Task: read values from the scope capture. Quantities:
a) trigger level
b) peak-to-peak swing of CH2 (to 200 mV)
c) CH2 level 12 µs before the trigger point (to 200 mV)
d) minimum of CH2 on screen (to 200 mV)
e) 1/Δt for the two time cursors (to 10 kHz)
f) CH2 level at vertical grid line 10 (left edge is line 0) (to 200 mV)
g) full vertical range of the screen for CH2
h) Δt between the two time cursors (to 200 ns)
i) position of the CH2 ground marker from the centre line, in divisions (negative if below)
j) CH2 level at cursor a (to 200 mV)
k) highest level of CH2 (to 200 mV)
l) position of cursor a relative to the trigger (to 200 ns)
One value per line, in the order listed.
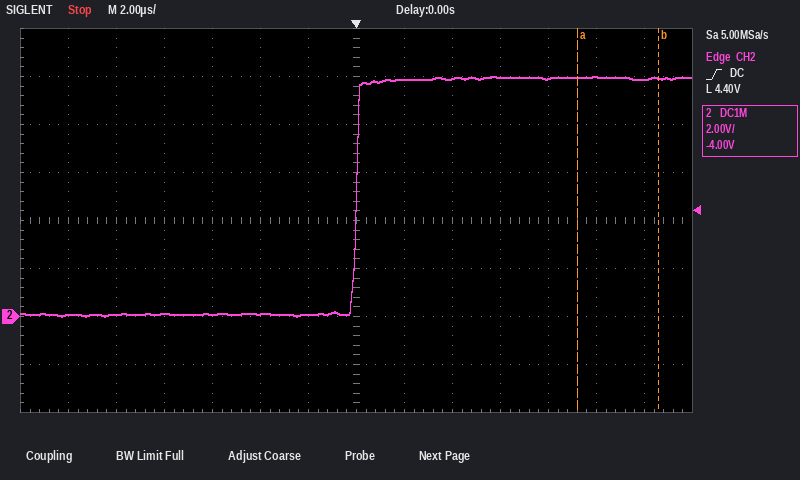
4.40 V
10.0 V
0.0 V
0.0 V
290 kHz
10.0 V
16 V
3.4 µs
-2.0 div
10.0 V
10.0 V
+9.2 µs
